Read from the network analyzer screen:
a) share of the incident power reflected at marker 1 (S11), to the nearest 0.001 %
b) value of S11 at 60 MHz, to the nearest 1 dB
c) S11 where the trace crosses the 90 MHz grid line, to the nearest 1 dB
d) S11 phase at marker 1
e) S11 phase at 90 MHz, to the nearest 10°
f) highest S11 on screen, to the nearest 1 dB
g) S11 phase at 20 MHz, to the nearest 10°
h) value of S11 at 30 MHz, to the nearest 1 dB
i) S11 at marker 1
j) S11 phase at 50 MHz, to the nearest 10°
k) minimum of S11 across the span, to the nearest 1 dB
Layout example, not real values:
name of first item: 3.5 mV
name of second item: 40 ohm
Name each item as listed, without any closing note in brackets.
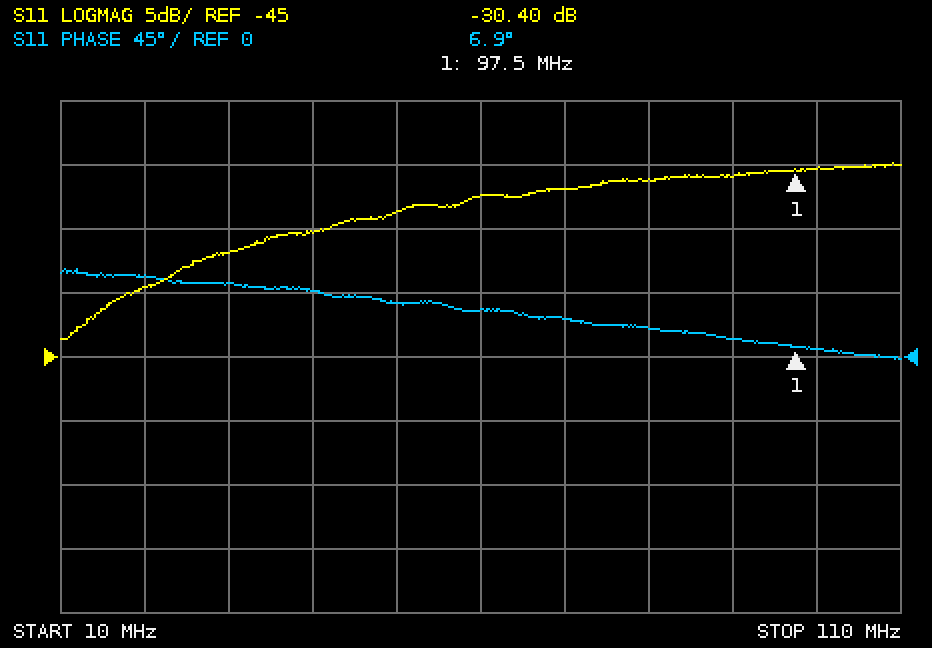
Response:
share of the incident power reflected at marker 1 (S11), to the nearest 0.001 %: 0.091 %
value of S11 at 60 MHz, to the nearest 1 dB: -32 dB
S11 where the trace crosses the 90 MHz grid line, to the nearest 1 dB: -31 dB
S11 phase at marker 1: 6.9°
S11 phase at 90 MHz, to the nearest 10°: 10°
highest S11 on screen, to the nearest 1 dB: -30 dB
S11 phase at 20 MHz, to the nearest 10°: 60°
value of S11 at 30 MHz, to the nearest 1 dB: -37 dB
S11 at marker 1: -30.40 dB
S11 phase at 50 MHz, to the nearest 10°: 40°
minimum of S11 across the span, to the nearest 1 dB: -44 dB
